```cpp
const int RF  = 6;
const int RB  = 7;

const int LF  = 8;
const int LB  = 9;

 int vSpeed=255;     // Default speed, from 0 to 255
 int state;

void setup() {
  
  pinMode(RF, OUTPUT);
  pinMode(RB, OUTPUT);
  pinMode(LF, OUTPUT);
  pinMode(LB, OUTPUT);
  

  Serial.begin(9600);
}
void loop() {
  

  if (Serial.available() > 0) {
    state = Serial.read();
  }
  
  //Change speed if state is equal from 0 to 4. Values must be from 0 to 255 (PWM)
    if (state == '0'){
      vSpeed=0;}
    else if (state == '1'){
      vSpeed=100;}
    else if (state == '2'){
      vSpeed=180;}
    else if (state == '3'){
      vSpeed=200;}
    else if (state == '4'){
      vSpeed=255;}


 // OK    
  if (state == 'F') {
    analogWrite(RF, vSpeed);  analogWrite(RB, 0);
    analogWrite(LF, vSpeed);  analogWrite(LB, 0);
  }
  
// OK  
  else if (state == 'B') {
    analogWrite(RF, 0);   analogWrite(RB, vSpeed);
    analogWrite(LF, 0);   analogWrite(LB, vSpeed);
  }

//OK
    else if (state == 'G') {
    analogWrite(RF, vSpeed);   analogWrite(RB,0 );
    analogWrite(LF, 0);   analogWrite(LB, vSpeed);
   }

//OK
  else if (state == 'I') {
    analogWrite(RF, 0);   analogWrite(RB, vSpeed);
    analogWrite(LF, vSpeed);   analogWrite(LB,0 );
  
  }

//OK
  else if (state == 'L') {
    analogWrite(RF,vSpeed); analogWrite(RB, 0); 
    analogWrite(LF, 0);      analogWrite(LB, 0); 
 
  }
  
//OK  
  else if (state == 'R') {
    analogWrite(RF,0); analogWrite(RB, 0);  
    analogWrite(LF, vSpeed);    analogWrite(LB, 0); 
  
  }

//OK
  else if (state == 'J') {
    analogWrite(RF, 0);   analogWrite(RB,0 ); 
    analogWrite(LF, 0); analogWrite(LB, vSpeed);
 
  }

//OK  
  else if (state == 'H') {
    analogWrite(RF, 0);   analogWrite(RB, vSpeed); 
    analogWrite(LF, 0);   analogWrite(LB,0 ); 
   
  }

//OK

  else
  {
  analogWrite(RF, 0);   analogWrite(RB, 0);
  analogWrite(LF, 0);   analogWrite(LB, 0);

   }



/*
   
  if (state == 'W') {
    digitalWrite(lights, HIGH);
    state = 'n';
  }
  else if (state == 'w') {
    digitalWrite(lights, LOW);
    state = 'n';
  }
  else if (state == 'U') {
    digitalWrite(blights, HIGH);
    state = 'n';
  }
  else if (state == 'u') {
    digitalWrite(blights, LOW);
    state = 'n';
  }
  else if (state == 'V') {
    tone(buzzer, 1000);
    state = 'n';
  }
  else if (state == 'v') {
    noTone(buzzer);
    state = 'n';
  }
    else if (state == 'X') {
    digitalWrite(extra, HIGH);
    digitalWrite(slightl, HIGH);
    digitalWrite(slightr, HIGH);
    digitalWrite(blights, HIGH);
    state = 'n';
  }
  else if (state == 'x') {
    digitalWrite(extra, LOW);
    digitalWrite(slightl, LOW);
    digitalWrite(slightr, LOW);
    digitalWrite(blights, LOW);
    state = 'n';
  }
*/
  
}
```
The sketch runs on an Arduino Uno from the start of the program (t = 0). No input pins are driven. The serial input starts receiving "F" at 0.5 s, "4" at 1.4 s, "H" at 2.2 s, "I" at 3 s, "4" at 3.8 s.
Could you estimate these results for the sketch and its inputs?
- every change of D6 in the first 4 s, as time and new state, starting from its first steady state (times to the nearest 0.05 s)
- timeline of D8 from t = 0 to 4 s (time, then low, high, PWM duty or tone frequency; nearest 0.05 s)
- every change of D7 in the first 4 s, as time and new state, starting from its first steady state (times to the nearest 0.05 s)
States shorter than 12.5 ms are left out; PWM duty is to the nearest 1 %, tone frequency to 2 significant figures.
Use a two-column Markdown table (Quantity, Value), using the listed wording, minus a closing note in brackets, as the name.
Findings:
| Quantity | Value |
|---|---|
| every change of D6 in the first 4 s, as time and new state, starting from its first steady state | 0 s low; 0.5 s high; 1.4 s low |
| timeline of D8 from t = 0 to 4 s | 0 s low; 0.5 s high; 1.4 s low; 3 s high; 3.8 s low |
| every change of D7 in the first 4 s, as time and new state, starting from its first steady state | 0 s low; 2.2 s high; 3.8 s low |
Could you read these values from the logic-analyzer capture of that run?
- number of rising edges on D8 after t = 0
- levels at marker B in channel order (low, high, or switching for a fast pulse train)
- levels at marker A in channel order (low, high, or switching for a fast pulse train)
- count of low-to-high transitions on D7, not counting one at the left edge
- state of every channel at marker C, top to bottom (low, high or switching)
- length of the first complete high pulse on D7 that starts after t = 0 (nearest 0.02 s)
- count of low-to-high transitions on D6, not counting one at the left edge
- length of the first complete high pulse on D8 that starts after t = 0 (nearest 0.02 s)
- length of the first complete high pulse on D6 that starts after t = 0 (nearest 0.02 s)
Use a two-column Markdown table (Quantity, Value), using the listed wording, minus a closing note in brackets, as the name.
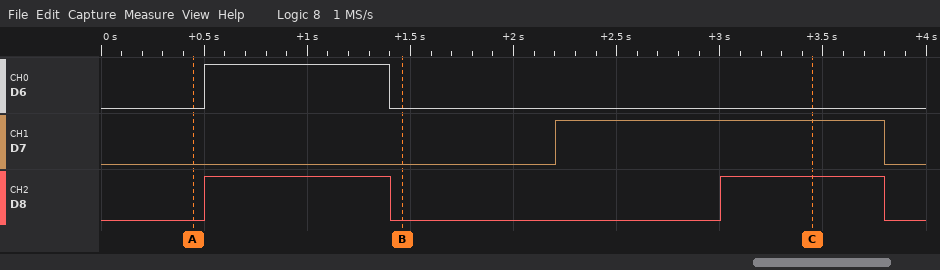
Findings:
| Quantity | Value |
|---|---|
| number of rising edges on D8 after t = 0 | 2 |
| levels at marker B in channel order | D6 low, D7 low, D8 low |
| levels at marker A in channel order | D6 low, D7 low, D8 low |
| count of low-to-high transitions on D7, not counting one at the left edge | 1 |
| state of every channel at marker C, top to bottom | D6 low, D7 high, D8 high |
| length of the first complete high pulse on D7 that starts after t = 0 | 1.60 s |
| count of low-to-high transitions on D6, not counting one at the left edge | 1 |
| length of the first complete high pulse on D8 that starts after t = 0 | 0.90 s |
| length of the first complete high pulse on D6 that starts after t = 0 | 0.90 s |
